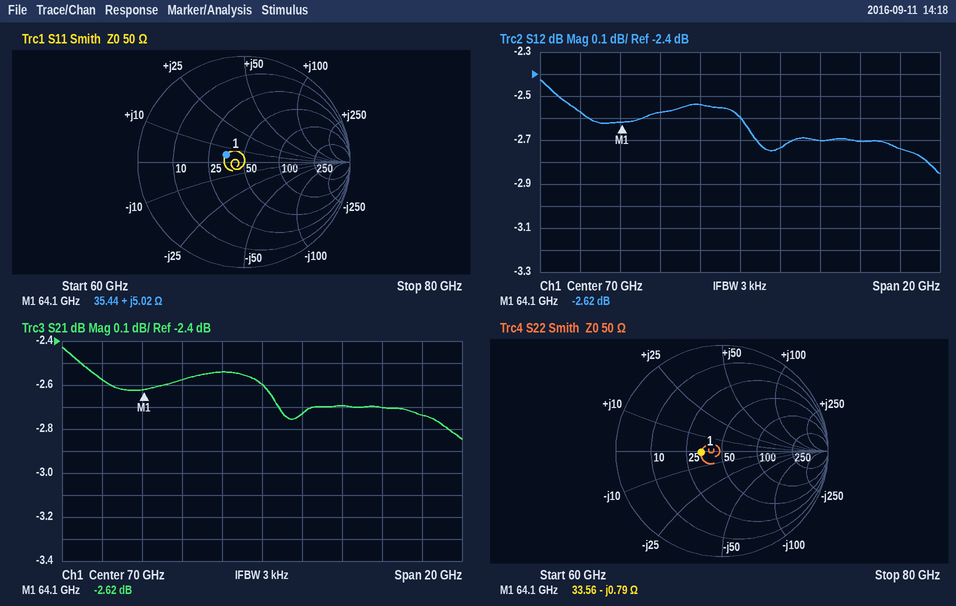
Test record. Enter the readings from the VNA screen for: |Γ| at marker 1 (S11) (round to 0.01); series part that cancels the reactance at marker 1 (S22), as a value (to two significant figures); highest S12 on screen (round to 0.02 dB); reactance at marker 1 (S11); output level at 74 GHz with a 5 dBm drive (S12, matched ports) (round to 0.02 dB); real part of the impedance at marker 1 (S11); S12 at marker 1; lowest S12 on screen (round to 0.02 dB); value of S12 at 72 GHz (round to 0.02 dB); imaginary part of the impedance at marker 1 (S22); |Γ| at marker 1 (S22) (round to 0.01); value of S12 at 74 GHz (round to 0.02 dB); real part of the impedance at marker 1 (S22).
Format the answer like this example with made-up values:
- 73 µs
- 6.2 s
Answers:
- 0.18
- 2.0 pH
- -2.42 dB
- +5.02 Ω
- 2.30 dBm
- 35.44 Ω
- -2.62 dB
- -2.86 dB
- -2.74 dB
- -0.79 Ω
- 0.20
- -2.70 dB
- 33.56 Ω
